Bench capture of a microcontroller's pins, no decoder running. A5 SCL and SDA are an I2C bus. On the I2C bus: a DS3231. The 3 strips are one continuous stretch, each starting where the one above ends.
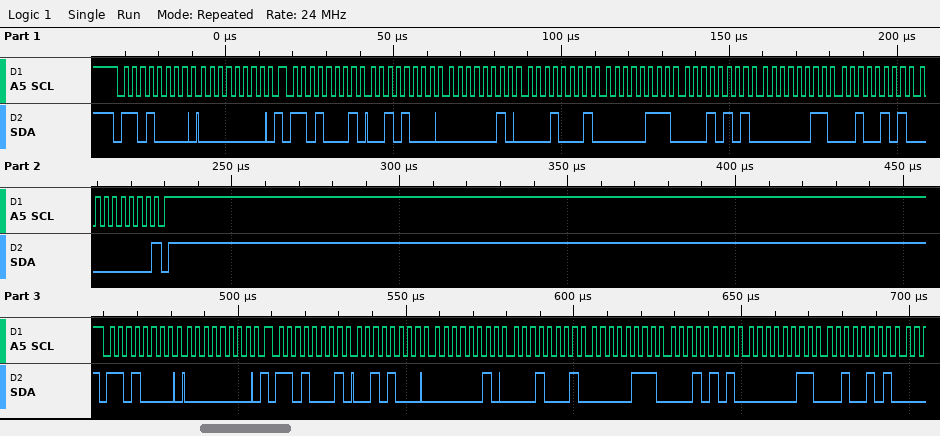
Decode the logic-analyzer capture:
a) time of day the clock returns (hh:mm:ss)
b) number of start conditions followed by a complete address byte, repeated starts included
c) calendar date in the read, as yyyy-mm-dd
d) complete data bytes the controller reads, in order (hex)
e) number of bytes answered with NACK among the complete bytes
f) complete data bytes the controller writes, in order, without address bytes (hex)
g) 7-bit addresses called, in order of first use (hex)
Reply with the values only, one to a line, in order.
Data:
11:02:28
4
2025-03-15
28 02 11 07 15 03 25 00 28 02 11 07 15 03 25
1
00 00
0x68
